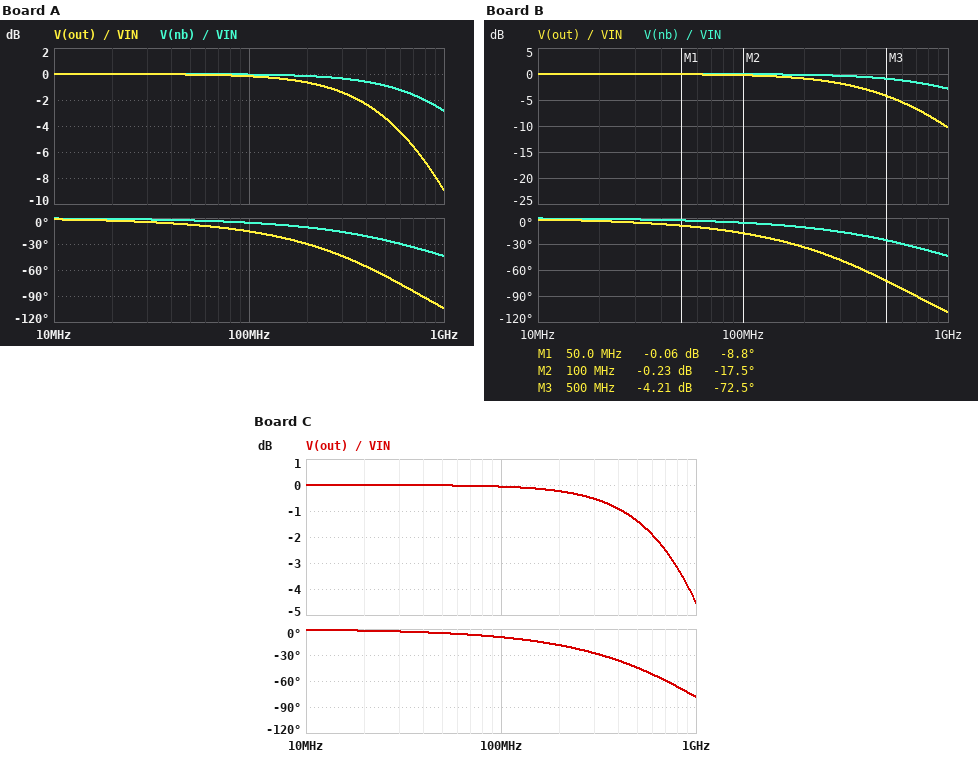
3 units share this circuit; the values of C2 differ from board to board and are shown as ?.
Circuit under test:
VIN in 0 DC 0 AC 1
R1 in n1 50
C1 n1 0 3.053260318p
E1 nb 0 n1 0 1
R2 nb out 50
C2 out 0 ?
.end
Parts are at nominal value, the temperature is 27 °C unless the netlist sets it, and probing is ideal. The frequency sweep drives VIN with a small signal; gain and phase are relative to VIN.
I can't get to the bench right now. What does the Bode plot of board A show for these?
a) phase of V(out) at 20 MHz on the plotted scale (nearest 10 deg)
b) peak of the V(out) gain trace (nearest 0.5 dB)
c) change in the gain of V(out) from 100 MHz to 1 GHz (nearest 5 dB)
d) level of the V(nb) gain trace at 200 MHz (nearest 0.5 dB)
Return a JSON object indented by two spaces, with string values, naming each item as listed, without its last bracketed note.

{
  "phase of V(out) at 20 MHz on the plotted scale": "0 deg",
  "peak of the V(out) gain trace": "0 dB",
  "change in the gain of V(out) from 100 MHz to 1 GHz": "-10 dB",
  "level of the V(nb) gain trace at 200 MHz": "0 dB"
}
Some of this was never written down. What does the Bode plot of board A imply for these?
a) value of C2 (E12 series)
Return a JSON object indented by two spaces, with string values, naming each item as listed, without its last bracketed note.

{
  "value of C2": "5.6 pF"
}
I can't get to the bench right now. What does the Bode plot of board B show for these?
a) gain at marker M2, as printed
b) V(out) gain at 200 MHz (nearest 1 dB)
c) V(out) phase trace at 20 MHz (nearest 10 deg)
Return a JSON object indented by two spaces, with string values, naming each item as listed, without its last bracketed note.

{
  "gain at marker M2, as printed": "-0.23 dB",
  "V(out) gain at 200 MHz": "-1 dB",
  "V(out) phase trace at 20 MHz": "0 deg"
}
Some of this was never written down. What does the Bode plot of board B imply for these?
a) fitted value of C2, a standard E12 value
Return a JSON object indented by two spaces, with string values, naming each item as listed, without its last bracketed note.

{
  "fitted value of C2, a standard E12 value": "6.8 pF"
}
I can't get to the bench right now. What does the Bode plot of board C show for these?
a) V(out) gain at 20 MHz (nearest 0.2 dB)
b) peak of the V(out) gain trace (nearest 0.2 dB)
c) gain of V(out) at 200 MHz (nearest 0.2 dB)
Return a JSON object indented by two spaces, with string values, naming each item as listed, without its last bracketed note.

{
  "V(out) gain at 20 MHz": "0 dB",
  "peak of the V(out) gain trace": "0 dB",
  "gain of V(out) at 200 MHz": "-0.2 dB"
}
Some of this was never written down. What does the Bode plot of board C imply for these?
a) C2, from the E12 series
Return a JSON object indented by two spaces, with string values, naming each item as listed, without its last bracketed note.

{
  "C2, from the E12 series": "2.2 pF"
}
